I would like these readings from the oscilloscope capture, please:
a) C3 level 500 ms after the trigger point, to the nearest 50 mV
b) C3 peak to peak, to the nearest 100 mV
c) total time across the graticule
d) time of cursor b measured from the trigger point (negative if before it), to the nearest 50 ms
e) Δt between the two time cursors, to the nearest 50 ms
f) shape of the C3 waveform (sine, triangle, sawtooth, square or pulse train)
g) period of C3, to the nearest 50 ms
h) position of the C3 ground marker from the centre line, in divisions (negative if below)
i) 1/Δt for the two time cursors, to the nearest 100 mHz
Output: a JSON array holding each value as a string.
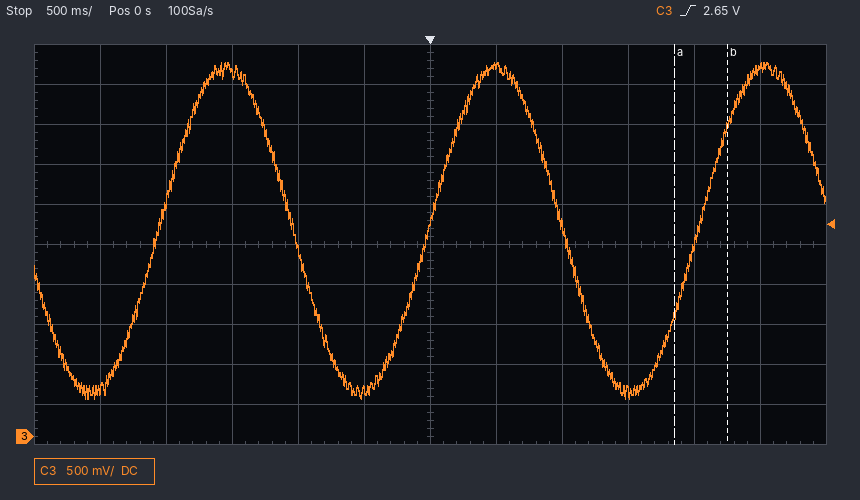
["4.65 V", "4.20 V", "6 s", "+2.25 s", "400 ms", "sine", "2.05 s", "-4.8 div", "2.5 Hz"]
